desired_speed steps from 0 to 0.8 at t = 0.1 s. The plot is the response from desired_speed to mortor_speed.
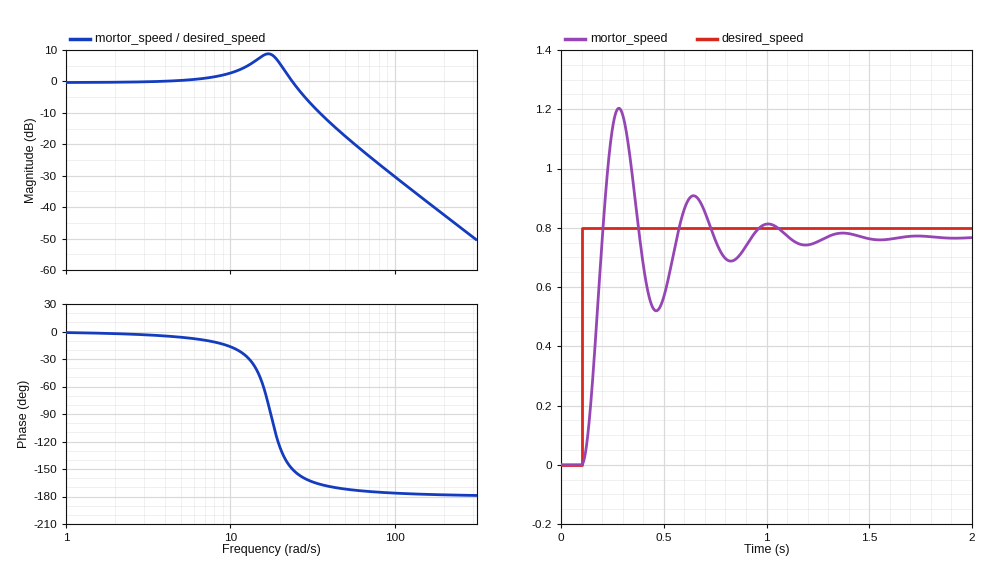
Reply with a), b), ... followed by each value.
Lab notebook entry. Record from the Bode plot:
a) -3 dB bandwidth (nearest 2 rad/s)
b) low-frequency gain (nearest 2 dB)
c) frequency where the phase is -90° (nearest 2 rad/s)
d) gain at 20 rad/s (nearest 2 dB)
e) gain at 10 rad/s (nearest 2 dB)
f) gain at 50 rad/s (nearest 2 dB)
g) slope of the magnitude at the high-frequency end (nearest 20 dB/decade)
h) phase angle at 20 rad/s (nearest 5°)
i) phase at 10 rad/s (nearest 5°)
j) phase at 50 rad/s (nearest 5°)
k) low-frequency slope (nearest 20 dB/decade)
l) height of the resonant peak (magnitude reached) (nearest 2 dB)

a) 26 rad/s
b) 0 dB
c) 18 rad/s
d) 6 dB
e) 2 dB
f) -18 dB
g) -40 dB/decade
h) -125°
i) -15°
j) -170°
k) 0 dB/decade
l) 8 dB
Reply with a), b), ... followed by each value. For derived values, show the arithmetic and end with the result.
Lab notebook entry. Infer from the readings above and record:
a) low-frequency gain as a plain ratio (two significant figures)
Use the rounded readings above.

a) 10^(0 / 20) = 1.0
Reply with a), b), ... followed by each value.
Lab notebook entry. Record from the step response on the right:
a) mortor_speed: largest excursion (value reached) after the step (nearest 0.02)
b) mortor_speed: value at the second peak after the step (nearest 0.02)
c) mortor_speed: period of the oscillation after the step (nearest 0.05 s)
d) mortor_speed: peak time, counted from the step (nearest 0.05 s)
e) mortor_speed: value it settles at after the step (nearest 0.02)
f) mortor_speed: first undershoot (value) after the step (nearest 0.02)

a) 1.20
b) 0.90
c) 0.35 s
d) 0.20 s
e) 0.76
f) 0.52
